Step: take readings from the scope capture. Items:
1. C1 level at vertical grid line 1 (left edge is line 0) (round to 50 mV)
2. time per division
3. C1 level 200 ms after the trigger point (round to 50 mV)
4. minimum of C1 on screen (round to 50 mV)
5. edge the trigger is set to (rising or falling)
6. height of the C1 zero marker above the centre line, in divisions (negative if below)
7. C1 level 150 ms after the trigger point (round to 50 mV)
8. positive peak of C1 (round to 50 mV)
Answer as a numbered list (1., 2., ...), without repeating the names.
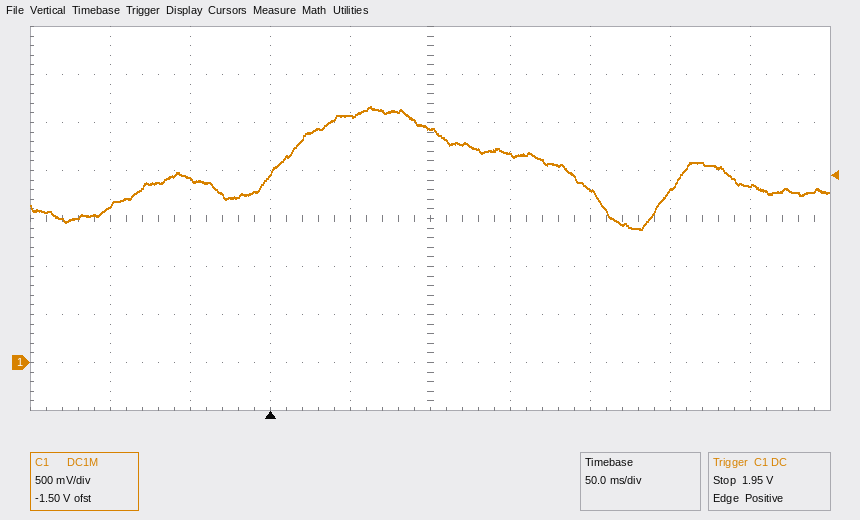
1. 1.65 V
2. 50 ms
3. 1.80 V
4. 1.40 V
5. rising
6. -3.0 div
7. 2.15 V
8. 2.65 V
